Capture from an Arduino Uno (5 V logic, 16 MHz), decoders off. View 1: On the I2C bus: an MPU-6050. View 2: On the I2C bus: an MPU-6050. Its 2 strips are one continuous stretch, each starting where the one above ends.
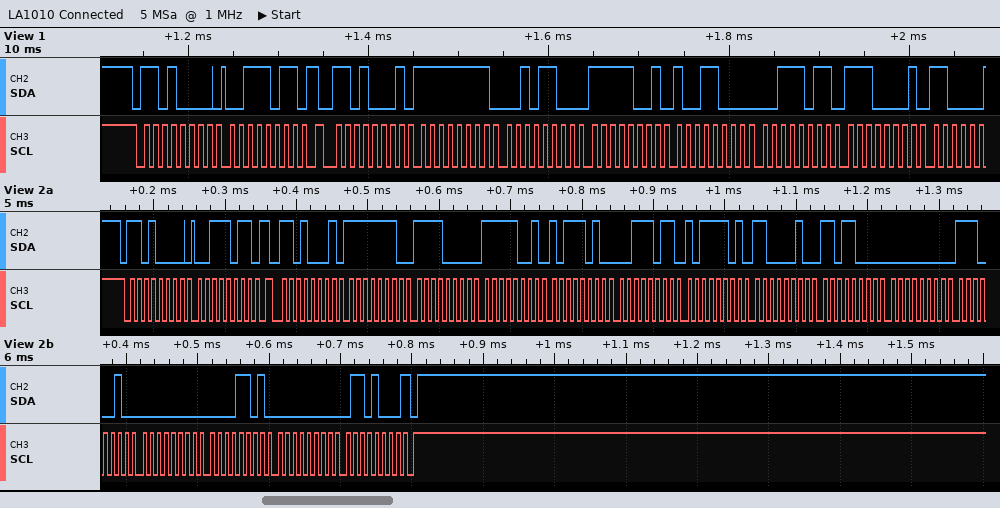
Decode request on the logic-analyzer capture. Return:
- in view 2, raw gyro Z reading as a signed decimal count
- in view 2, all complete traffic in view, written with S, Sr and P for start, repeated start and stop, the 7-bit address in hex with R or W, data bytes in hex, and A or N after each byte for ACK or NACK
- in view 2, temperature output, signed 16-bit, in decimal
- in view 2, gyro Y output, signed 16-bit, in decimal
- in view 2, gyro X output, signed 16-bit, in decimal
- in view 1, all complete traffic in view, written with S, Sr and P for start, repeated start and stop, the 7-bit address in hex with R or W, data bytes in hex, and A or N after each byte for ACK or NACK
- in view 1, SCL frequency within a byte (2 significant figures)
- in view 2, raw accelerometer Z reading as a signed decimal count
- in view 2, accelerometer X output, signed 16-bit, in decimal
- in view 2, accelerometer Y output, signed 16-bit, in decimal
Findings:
104
S 68W A 3B A Sr 68R A FE A F0 A F9 A BA A 3B A BD A C2 A D8 A 00 A E2 A 00 A 0D A 00 A 68 N P
-15656
13
226
S 68W A 3B A Sr 68R A FF A 2C A F9 A 98 A 3B A E1 A
100 kHz
15293
-272
-1606
